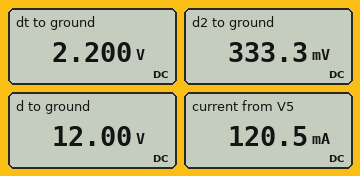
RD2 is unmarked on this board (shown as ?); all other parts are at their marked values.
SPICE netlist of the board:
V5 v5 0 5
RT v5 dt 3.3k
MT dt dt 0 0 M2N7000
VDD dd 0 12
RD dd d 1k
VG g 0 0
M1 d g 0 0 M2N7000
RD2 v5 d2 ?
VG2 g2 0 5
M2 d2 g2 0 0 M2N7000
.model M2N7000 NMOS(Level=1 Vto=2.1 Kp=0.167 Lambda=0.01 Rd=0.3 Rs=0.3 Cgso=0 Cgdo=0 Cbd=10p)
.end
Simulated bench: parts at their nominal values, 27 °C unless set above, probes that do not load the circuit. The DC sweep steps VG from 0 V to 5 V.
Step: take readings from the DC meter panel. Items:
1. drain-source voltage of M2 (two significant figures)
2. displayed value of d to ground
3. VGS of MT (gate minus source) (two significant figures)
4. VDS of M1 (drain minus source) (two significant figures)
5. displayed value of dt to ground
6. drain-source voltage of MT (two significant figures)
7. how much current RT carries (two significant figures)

330 mV
12.00 V
2.2 V
12 V
2.200 V
2.2 V
850 µA
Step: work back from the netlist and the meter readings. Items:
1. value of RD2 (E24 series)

39 Ω
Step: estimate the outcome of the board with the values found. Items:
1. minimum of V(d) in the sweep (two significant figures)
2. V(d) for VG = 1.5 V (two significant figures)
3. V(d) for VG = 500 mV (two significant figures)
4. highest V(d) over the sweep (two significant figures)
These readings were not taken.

32 mV
12 V
12 V
12 V
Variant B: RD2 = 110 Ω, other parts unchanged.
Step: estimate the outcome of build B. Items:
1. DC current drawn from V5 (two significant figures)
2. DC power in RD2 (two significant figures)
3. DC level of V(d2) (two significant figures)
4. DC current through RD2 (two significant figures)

45 mA
220 mW
120 mV
44 mA
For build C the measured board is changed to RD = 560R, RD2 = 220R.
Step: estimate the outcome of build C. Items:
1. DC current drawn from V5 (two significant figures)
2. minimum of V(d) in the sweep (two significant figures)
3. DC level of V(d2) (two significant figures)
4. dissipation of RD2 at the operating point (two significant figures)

23 mA
57 mV
60 mV
110 mW
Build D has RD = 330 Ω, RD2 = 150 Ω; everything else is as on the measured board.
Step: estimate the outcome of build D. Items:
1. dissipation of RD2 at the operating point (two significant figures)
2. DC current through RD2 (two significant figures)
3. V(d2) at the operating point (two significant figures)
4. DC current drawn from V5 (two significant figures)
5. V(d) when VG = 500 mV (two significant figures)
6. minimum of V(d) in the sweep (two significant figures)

160 mW
33 mA
88 mV
34 mA
12 V
97 mV
